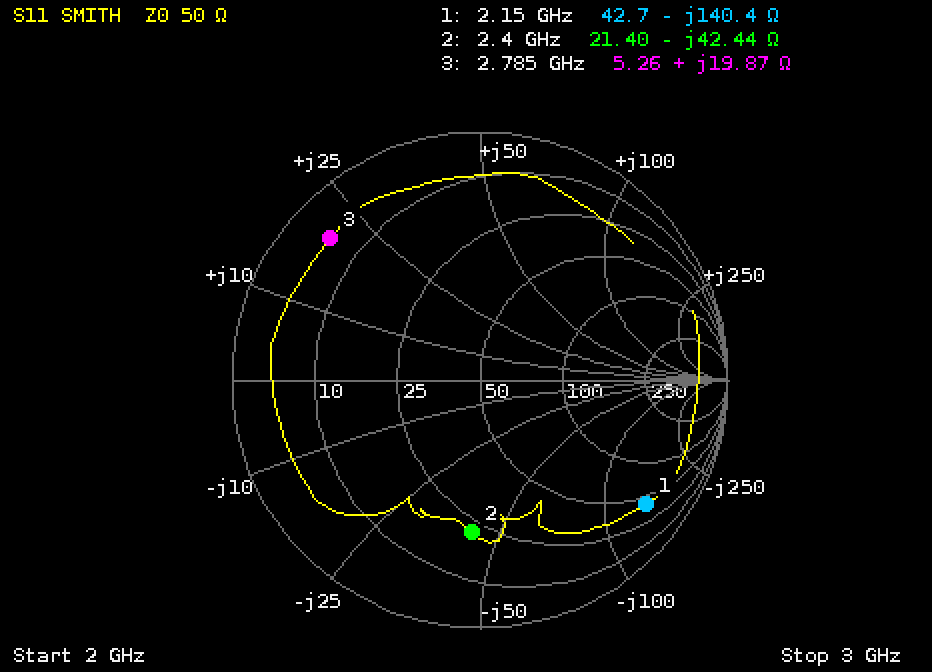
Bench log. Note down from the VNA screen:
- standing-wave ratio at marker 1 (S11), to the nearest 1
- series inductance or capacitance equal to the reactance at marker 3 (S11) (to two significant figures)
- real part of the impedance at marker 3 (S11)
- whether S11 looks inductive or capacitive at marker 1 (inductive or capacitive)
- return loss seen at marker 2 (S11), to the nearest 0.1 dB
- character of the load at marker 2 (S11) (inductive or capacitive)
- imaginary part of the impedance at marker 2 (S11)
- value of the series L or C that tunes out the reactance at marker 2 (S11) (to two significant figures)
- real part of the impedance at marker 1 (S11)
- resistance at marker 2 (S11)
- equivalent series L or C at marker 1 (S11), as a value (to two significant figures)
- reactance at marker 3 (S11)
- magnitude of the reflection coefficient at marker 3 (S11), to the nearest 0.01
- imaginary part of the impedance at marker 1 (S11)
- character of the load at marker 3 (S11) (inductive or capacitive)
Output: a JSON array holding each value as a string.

["11", "1.1 nH", "5.26 Ω", "capacitive", "4.2 dB", "capacitive", "-42.44 Ω", "2.8 nH", "42.7 Ω", "21.40 Ω", "530 fF", "+19.87 Ω", "0.83", "-140.4 Ω", "inductive"]
